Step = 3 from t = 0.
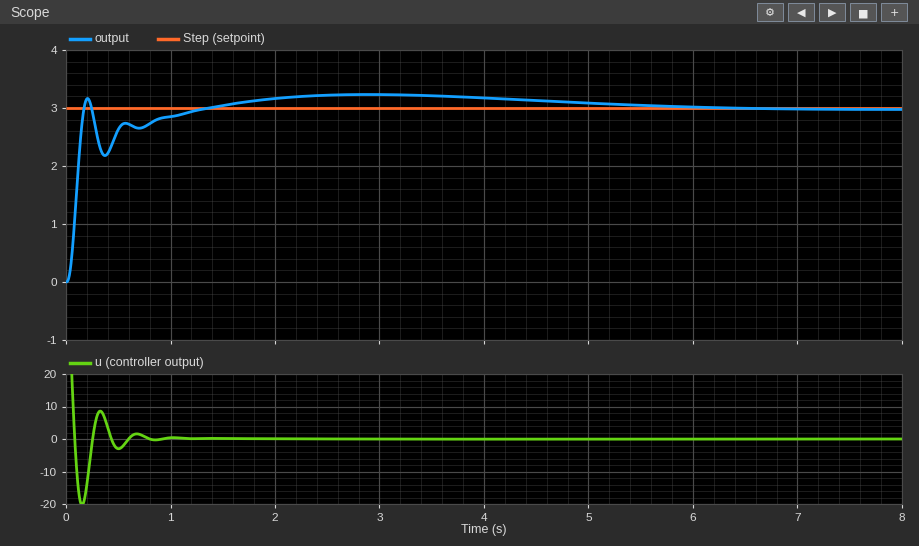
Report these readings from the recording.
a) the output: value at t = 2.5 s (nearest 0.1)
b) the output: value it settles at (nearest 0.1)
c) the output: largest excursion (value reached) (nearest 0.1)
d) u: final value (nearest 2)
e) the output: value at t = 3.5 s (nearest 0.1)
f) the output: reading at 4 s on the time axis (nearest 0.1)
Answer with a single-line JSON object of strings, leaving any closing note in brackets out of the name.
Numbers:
{"the output: value at t = 2.5 s": "3.2", "the output: value it settles at": "3.0", "the output: largest excursion (value reached)": "3.2", "u: final value": "0", "the output: value at t = 3.5 s": "3.2", "the output: reading at 4 s on the time axis": "3.2"}
